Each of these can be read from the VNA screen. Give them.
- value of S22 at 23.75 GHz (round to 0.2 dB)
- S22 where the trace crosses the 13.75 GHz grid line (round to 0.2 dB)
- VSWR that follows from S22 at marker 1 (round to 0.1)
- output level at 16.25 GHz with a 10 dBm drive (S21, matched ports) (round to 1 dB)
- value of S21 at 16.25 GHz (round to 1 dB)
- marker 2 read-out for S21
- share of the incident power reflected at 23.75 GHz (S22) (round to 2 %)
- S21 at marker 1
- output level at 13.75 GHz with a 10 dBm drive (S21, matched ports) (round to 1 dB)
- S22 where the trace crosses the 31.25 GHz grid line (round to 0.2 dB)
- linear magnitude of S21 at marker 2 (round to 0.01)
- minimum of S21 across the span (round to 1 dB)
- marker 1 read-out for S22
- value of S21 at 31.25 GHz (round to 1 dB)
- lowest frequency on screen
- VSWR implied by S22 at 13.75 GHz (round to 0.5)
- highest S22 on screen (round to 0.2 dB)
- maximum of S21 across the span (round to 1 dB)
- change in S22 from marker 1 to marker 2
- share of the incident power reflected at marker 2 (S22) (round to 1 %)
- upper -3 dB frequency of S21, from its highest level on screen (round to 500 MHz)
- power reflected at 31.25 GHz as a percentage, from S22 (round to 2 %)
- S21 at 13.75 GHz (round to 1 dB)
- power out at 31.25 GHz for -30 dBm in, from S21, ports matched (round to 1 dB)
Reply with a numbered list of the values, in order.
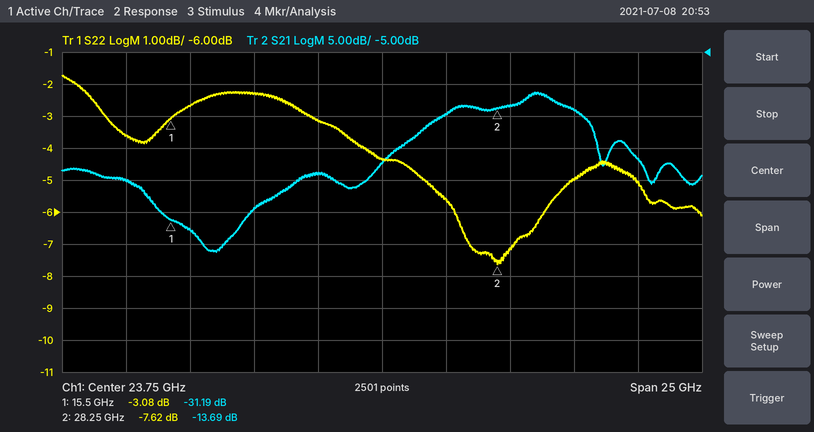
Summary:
1. -4.4 dB
2. -3.6 dB
3. 5.7
4. -23 dBm
5. -33 dB
6. -13.69 dB
7. 36 %
8. -31.19 dB
9. -15 dBm
10. -5.0 dB
11. 0.21
12. -36 dB
13. -3.08 dB
14. -14 dB
15. 11.25 GHz
16. 5.0
17. -1.8 dB
18. -11 dB
19. -4.54 dB
20. 17 %
21. 31.5 GHz
22. 32 %
23. -25 dB
24. -44 dBm
